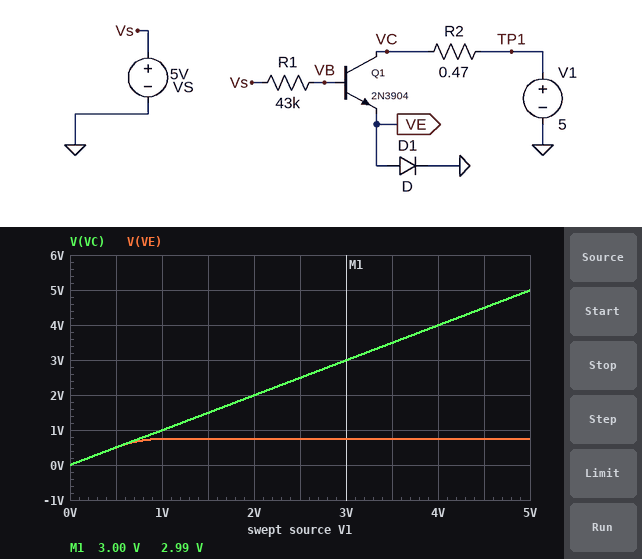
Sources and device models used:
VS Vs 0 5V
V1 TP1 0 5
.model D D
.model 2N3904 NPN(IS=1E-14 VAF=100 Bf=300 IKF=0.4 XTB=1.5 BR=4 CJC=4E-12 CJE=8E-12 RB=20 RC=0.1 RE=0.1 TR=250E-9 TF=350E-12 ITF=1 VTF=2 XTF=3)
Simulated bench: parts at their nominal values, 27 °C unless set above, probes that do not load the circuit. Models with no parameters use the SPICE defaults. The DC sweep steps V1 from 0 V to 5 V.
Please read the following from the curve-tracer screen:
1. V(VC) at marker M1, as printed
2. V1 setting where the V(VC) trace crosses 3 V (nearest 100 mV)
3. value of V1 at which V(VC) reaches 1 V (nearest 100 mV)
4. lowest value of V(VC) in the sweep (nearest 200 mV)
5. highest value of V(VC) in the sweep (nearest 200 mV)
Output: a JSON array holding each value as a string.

["2.99 V", "3.0 V", "1.0 V", "0 V", "5.0 V"]
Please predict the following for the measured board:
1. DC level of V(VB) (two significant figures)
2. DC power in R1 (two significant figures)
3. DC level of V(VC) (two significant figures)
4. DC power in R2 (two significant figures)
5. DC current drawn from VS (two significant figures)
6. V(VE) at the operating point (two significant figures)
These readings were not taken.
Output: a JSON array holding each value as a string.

["1.5 V", "290 µW", "5.0 V", "270 µW", "82 µA", "740 mV"]
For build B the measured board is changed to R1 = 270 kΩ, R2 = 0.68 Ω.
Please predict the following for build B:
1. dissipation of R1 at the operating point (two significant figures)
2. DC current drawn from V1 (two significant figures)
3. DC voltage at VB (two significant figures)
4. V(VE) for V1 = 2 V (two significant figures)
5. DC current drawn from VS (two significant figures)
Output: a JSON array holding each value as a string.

["48 µW", "4.1 mA", "1.4 V", "690 mV", "13 µA"]
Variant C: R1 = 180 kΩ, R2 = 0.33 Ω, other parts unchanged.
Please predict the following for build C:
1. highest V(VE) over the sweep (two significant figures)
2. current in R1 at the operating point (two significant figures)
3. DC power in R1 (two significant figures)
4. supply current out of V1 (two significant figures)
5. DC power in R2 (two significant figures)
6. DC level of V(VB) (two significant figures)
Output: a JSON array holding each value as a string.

["700 mV", "20 µA", "72 µW", "6.1 mA", "12 µW", "1.4 V"]
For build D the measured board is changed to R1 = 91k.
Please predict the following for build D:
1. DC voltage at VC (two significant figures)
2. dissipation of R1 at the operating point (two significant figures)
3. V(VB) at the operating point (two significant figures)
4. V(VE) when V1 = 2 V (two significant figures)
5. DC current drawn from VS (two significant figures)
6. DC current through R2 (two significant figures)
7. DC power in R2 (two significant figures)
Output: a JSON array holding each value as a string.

["5.0 V", "140 µW", "1.4 V", "720 mV", "39 µA", "12 mA", "66 µW"]
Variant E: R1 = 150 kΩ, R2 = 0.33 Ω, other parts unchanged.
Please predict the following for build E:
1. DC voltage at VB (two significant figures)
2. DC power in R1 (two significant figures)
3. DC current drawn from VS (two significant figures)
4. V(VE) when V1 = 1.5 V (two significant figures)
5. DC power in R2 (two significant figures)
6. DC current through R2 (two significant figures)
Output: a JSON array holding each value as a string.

["1.4 V", "86 µW", "24 µA", "710 mV", "18 µW", "7.3 mA"]
